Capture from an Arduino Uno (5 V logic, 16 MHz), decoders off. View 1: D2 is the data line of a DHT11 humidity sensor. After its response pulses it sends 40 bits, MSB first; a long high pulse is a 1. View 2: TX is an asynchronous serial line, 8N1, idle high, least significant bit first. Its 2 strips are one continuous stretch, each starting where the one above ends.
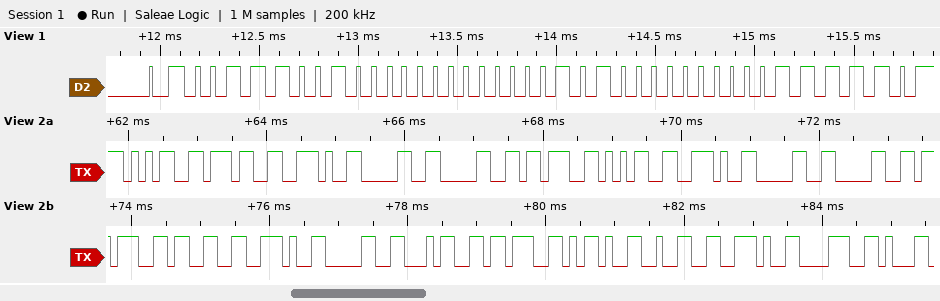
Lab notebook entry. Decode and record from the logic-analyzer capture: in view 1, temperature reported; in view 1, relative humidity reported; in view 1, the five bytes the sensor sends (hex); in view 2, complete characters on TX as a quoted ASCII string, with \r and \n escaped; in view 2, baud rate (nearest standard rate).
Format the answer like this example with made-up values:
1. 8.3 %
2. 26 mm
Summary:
1. 5.0 °C
2. 57 %
3. 39 00 05 00 3E
4. "57.00;5.00;3.04;-2.8"
5. 9600 baud
